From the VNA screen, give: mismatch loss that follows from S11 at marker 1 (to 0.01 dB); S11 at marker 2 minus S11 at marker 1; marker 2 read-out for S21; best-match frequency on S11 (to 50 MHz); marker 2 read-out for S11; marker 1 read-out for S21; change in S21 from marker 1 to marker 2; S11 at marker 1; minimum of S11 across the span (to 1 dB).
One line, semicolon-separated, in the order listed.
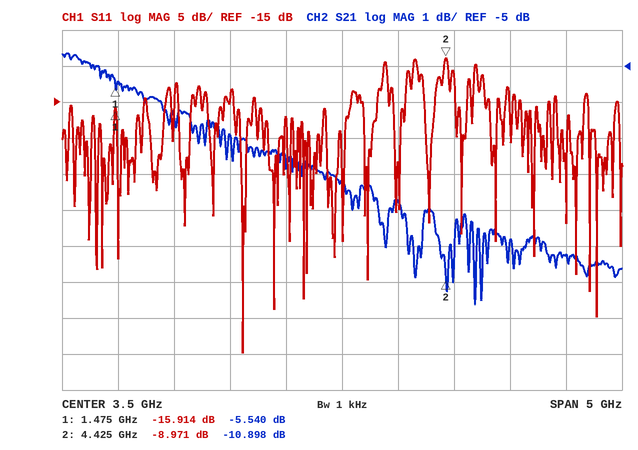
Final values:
0.11 dB; 6.943 dB; -10.898 dB; 2.60 GHz; -8.971 dB; -5.540 dB; -5.358 dB; -15.914 dB; -50 dB
